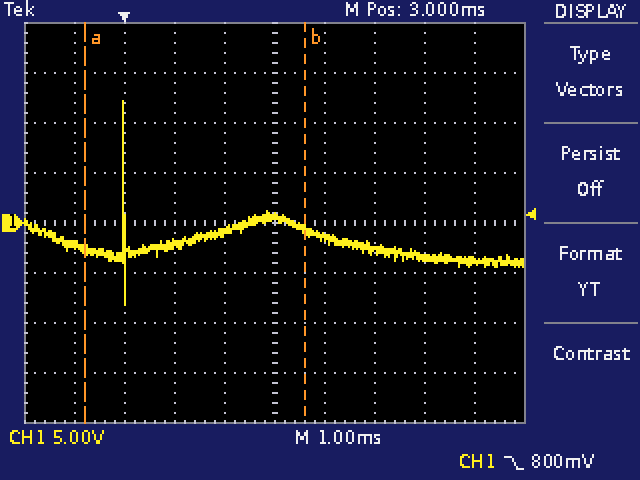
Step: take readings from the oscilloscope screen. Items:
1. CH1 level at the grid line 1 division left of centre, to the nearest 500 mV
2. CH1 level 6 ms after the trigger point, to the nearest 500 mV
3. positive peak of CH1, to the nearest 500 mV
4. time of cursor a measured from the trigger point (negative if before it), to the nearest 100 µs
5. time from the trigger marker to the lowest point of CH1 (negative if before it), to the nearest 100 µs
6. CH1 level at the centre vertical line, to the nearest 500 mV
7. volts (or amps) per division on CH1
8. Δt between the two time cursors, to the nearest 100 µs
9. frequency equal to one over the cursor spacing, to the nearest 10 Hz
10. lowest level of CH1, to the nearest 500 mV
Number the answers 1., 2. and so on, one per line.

1. -1.0 V
2. -3.5 V
3. 12.0 V
4. -800 µs
5. 0.0 ms
6. 500 mV
7. 5 V
8. 4.4 ms
9. 230 Hz
10. -8.0 V
